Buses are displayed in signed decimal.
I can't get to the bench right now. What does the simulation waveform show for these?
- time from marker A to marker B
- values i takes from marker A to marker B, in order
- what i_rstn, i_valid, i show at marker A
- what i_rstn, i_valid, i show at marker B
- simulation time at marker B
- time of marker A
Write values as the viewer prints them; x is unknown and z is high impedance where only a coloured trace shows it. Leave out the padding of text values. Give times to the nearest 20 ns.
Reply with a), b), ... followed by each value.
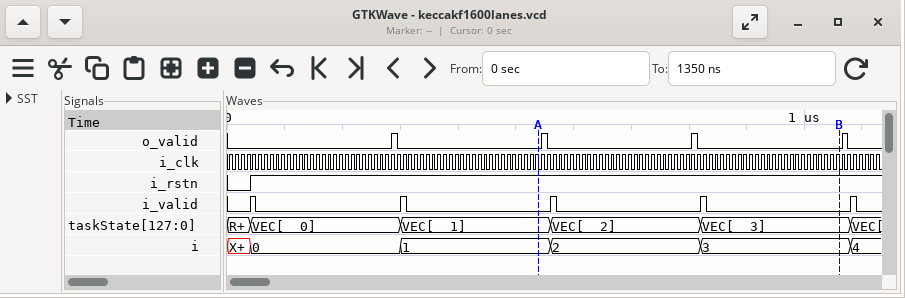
a) 520 ns
b) 1, 2, 3
c) i_rstn=1, i_valid=0, i=1
d) i_rstn=1, i_valid=0, i=3
e) 1060 ns
f) 540 ns
